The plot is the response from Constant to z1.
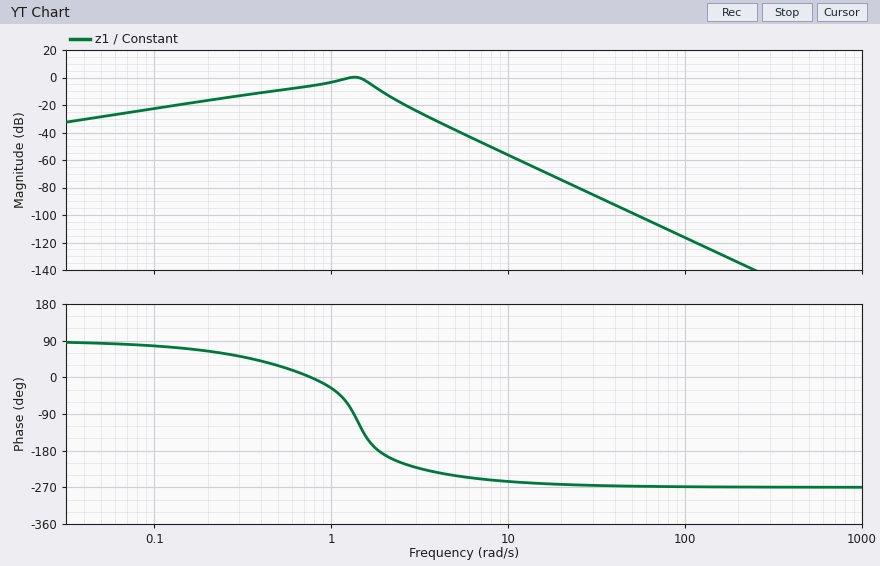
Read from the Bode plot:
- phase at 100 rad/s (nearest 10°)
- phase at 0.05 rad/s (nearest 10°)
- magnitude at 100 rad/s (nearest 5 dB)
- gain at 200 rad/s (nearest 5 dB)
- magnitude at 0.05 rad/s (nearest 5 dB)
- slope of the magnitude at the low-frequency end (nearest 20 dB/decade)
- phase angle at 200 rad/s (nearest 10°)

-270°
80°
-115 dB
-135 dB
-30 dB
20 dB/decade
-270°
